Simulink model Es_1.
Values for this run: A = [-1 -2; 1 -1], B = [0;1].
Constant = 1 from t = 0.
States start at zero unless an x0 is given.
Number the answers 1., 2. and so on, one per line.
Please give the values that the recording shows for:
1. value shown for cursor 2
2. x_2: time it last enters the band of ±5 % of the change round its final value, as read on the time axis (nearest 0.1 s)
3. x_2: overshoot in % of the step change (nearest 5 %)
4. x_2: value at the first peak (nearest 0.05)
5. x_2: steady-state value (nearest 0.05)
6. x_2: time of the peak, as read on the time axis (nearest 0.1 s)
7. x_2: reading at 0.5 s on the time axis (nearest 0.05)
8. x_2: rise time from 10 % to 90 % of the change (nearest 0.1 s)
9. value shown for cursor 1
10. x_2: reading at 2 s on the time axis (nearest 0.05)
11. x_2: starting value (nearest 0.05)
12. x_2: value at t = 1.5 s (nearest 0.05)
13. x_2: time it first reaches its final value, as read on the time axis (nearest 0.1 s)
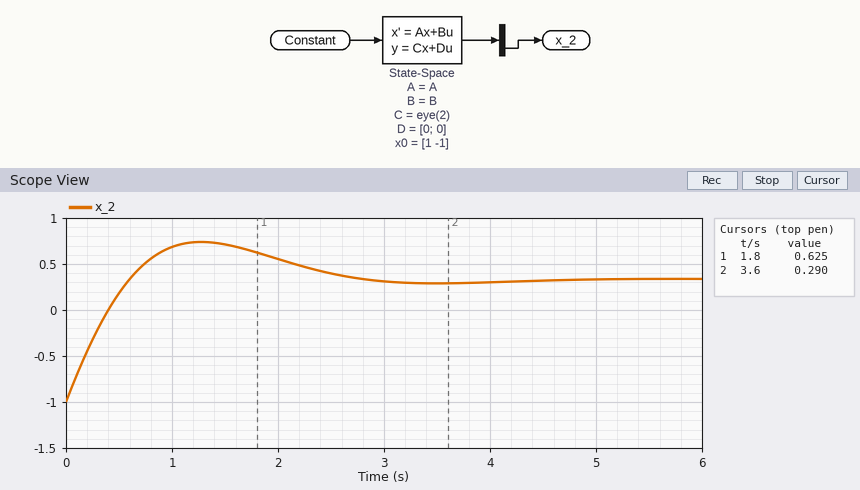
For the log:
1. 0.290
2. 2.5 s
3. 30 %
4. 0.75
5. 0.35
6. 1.3 s
7. 0.20
8. 0.5 s
9. 0.625
10. 0.55
11. -1.00
12. 0.70
13. 0.6 s
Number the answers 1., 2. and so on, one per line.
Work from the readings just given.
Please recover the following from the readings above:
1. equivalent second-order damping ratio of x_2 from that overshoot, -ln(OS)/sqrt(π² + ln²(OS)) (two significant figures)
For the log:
1. 0.36
